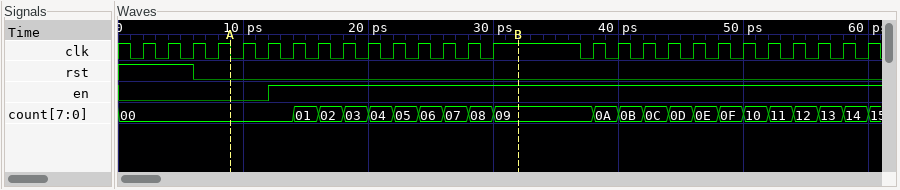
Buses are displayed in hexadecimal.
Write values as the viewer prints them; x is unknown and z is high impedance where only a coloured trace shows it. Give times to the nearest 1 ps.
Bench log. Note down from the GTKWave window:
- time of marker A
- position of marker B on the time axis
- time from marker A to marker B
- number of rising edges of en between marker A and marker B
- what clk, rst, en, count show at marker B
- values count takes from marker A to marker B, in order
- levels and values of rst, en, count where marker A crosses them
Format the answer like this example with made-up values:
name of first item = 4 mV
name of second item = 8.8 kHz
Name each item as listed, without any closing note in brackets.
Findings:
time of marker A = 9 ps
position of marker B on the time axis = 32 ps
time from marker A to marker B = 23 ps
number of rising edges of en between marker A and marker B = 1
what clk, rst, en, count show at marker B = clk=1, rst=0, en=1, count=09
values count takes from marker A to marker B, in order = 00, 01, 02, 03, 04, 05, 06, 07, 08, 09
levels and values of rst, en, count where marker A crosses them = rst=0, en=0, count=00
